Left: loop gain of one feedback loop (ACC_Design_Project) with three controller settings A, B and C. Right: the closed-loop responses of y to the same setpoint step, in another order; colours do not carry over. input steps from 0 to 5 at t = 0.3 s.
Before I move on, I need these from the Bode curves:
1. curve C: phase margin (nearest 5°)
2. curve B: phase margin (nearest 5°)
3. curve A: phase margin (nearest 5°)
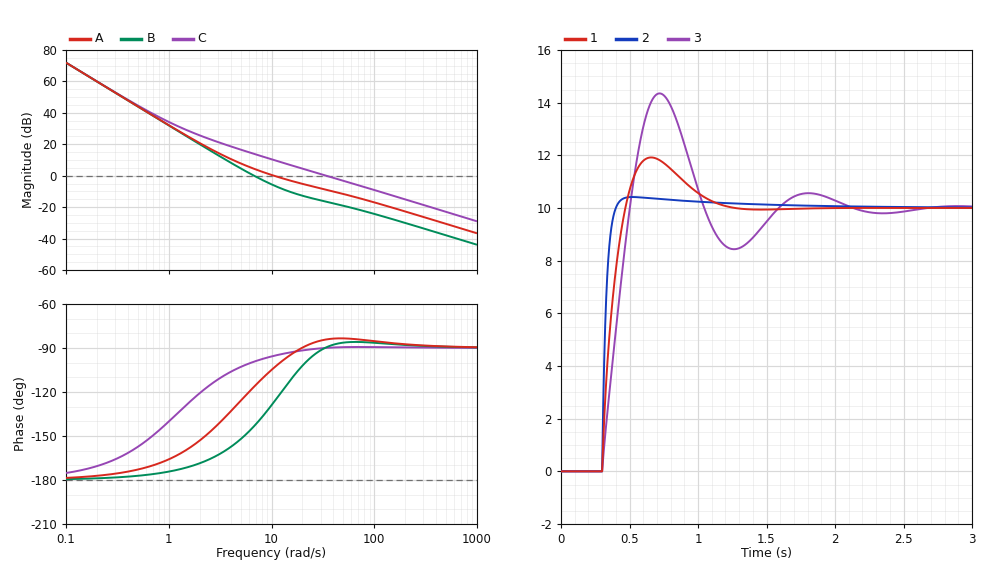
90°
35°
75°
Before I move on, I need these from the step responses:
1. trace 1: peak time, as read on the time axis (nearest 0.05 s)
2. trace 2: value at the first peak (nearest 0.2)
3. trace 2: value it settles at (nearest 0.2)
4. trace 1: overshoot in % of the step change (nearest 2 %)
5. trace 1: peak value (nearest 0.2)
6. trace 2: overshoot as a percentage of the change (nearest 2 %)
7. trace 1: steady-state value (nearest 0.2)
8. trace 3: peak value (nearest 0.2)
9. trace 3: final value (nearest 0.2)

0.65 s
10.4
10.0
20 %
12.0
4 %
10.0
14.4
10.0
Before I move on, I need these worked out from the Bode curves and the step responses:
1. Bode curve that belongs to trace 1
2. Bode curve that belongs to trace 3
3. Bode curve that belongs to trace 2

A
B
C
